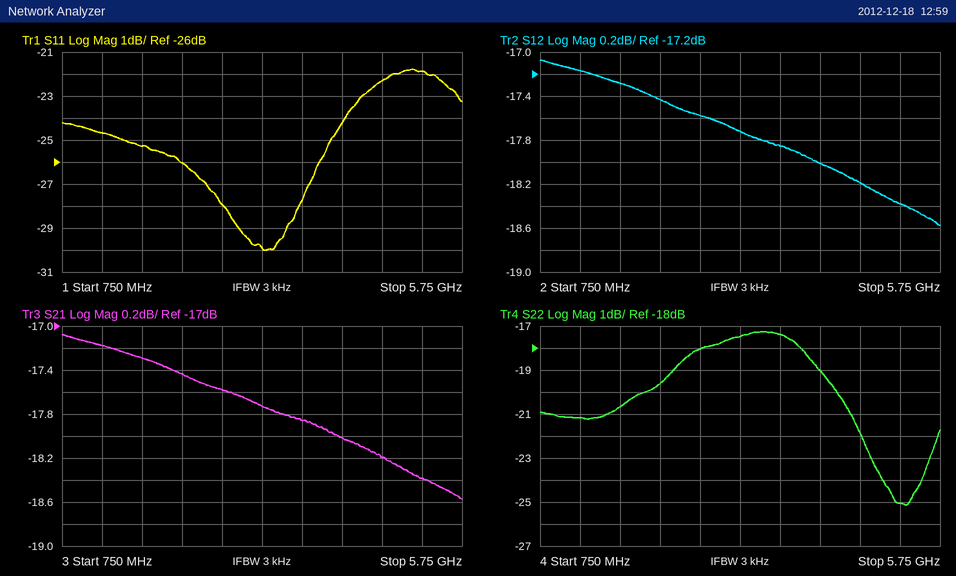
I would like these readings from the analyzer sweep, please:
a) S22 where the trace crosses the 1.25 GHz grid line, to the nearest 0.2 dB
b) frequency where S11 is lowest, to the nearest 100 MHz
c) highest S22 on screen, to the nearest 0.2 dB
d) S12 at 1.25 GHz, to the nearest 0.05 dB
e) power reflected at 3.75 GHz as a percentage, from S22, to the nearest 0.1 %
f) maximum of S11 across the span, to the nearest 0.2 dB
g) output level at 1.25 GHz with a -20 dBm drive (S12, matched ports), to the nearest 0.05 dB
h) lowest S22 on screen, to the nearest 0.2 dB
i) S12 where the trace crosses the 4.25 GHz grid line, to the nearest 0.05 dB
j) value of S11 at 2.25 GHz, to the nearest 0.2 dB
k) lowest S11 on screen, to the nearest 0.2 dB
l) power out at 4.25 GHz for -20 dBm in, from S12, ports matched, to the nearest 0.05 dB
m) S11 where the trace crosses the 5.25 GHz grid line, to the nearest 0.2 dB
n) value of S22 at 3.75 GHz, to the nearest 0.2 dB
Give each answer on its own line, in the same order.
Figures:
-21.2 dB
3.3 GHz
-17.2 dB
-17.15 dB
1.8 %
-21.8 dB
-37.15 dBm
-25.2 dB
-18.00 dB
-26.0 dB
-30.0 dB
-38.00 dBm
-21.8 dB
-17.4 dB
